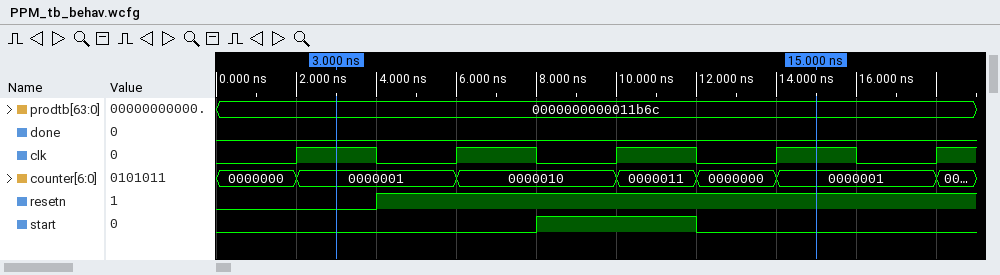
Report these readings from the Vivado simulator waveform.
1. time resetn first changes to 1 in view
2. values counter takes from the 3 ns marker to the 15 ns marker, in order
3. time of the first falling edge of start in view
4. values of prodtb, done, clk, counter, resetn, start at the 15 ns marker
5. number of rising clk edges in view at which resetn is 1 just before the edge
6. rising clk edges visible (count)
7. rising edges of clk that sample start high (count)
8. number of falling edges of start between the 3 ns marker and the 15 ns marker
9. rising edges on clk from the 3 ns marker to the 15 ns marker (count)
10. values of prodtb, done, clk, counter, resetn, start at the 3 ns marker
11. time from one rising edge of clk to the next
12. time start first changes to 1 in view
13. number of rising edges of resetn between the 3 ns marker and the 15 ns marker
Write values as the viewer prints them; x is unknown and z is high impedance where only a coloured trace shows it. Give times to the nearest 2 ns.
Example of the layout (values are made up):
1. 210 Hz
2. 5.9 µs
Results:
1. 4 ns
2. 0000001, 0000010, 0000011, 0000000, 0000001
3. 12 ns
4. prodtb=0000000000011b6c, done=0, clk=1, counter=0000001, resetn=1, start=0
5. 4
6. 5
7. 1
8. 1
9. 3
10. prodtb=0000000000011b6c, done=0, clk=1, counter=0000001, resetn=0, start=0
11. 4 ns
12. 8 ns
13. 1
